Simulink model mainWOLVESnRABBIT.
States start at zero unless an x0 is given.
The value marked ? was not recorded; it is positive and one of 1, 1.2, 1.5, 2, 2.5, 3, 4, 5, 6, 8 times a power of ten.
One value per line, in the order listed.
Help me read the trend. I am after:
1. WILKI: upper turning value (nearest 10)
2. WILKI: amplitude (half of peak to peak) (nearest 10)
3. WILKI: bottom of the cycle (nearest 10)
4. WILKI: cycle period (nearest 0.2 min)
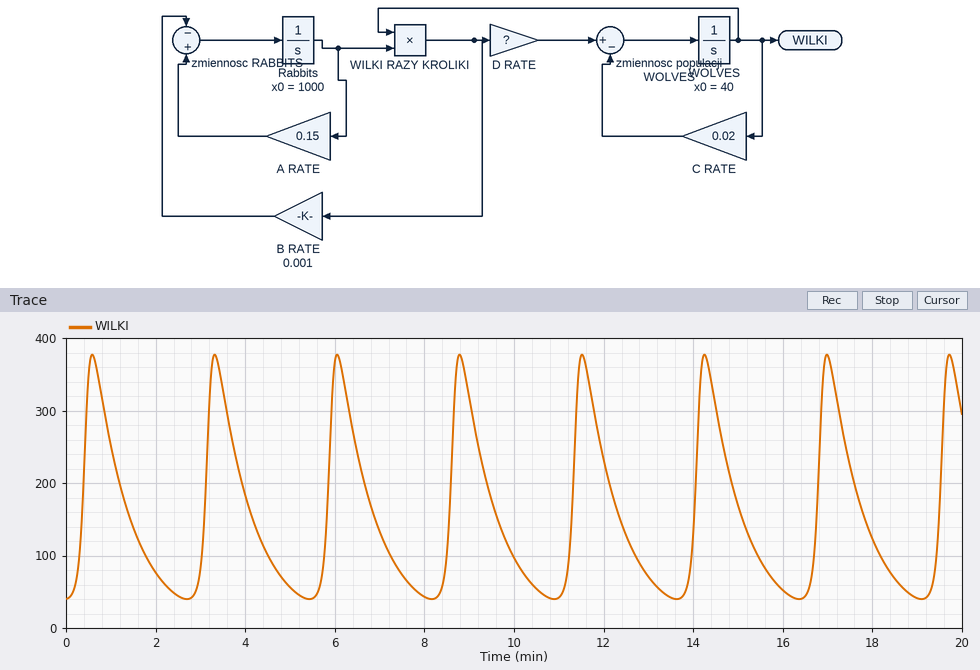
380
170
40
2.8 min
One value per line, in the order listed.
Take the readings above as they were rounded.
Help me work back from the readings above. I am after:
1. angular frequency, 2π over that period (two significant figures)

2.2 rad/min
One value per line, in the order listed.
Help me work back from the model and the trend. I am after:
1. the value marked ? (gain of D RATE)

2.5e-05
